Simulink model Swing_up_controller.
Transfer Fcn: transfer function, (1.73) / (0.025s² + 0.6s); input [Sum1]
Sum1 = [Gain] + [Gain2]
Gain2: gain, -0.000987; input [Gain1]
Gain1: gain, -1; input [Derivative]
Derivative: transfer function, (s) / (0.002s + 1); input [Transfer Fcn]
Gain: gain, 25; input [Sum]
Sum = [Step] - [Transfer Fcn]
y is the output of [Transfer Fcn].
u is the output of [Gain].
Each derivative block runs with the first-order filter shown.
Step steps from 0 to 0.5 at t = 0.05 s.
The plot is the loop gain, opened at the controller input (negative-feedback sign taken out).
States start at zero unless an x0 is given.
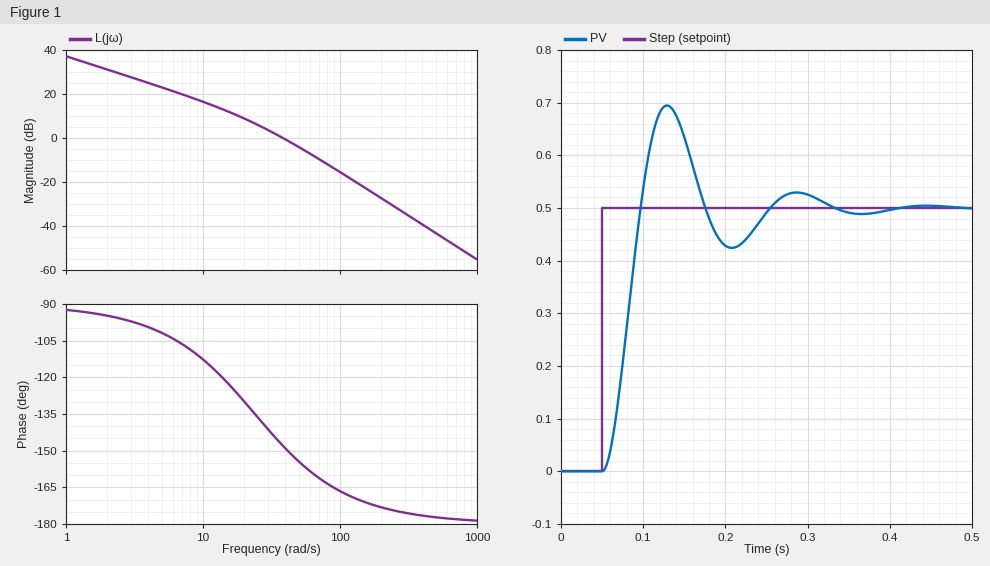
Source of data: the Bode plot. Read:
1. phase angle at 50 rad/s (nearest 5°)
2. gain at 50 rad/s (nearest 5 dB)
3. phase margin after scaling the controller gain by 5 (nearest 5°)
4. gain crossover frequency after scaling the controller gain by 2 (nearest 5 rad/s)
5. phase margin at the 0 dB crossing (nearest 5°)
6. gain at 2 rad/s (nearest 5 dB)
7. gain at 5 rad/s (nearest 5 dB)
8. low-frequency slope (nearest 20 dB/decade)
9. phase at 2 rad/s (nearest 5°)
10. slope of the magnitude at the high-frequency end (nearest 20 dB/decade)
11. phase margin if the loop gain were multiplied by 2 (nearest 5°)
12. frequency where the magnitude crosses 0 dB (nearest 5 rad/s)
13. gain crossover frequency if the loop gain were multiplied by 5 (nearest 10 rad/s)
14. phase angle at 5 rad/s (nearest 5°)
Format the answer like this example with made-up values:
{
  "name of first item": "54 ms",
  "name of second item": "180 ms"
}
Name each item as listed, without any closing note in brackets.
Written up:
{
  "phase angle at 50 rad/s": "-155°",
  "gain at 50 rad/s": "-5 dB",
  "phase margin after scaling the controller gain by 5": "15°",
  "gain crossover frequency after scaling the controller gain by 2": "55 rad/s",
  "phase margin at the 0 dB crossing": "30°",
  "gain at 2 rad/s": "30 dB",
  "gain at 5 rad/s": "25 dB",
  "low-frequency slope": "-20 dB/decade",
  "phase at 2 rad/s": "-95°",
  "slope of the magnitude at the high-frequency end": "-40 dB/decade",
  "phase margin if the loop gain were multiplied by 2": "25°",
  "frequency where the magnitude crosses 0 dB": "40 rad/s",
  "gain crossover frequency if the loop gain were multiplied by 5": "90 rad/s",
  "phase angle at 5 rad/s": "-100°"
}
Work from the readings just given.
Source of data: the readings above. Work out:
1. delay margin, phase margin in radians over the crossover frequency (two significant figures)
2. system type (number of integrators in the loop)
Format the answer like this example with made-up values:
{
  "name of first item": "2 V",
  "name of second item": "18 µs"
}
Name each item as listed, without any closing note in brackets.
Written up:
{
  "delay margin, phase margin in radians over the crossover frequency": "0.013 s",
  "system type": "1"
}
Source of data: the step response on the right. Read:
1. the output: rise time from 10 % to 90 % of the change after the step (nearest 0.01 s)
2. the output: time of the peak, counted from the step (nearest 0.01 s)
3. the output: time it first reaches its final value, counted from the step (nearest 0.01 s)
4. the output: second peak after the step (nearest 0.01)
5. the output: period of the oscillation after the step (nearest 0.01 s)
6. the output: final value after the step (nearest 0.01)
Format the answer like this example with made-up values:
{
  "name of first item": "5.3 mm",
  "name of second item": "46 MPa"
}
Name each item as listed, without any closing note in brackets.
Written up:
{
  "the output: rise time from 10 % to 90 % of the change after the step": "0.03 s",
  "the output: time of the peak, counted from the step": "0.08 s",
  "the output: time it first reaches its final value, counted from the step": "0.05 s",
  "the output: second peak after the step": "0.53",
  "the output: period of the oscillation after the step": "0.16 s",
  "the output: final value after the step": "0.50"
}
